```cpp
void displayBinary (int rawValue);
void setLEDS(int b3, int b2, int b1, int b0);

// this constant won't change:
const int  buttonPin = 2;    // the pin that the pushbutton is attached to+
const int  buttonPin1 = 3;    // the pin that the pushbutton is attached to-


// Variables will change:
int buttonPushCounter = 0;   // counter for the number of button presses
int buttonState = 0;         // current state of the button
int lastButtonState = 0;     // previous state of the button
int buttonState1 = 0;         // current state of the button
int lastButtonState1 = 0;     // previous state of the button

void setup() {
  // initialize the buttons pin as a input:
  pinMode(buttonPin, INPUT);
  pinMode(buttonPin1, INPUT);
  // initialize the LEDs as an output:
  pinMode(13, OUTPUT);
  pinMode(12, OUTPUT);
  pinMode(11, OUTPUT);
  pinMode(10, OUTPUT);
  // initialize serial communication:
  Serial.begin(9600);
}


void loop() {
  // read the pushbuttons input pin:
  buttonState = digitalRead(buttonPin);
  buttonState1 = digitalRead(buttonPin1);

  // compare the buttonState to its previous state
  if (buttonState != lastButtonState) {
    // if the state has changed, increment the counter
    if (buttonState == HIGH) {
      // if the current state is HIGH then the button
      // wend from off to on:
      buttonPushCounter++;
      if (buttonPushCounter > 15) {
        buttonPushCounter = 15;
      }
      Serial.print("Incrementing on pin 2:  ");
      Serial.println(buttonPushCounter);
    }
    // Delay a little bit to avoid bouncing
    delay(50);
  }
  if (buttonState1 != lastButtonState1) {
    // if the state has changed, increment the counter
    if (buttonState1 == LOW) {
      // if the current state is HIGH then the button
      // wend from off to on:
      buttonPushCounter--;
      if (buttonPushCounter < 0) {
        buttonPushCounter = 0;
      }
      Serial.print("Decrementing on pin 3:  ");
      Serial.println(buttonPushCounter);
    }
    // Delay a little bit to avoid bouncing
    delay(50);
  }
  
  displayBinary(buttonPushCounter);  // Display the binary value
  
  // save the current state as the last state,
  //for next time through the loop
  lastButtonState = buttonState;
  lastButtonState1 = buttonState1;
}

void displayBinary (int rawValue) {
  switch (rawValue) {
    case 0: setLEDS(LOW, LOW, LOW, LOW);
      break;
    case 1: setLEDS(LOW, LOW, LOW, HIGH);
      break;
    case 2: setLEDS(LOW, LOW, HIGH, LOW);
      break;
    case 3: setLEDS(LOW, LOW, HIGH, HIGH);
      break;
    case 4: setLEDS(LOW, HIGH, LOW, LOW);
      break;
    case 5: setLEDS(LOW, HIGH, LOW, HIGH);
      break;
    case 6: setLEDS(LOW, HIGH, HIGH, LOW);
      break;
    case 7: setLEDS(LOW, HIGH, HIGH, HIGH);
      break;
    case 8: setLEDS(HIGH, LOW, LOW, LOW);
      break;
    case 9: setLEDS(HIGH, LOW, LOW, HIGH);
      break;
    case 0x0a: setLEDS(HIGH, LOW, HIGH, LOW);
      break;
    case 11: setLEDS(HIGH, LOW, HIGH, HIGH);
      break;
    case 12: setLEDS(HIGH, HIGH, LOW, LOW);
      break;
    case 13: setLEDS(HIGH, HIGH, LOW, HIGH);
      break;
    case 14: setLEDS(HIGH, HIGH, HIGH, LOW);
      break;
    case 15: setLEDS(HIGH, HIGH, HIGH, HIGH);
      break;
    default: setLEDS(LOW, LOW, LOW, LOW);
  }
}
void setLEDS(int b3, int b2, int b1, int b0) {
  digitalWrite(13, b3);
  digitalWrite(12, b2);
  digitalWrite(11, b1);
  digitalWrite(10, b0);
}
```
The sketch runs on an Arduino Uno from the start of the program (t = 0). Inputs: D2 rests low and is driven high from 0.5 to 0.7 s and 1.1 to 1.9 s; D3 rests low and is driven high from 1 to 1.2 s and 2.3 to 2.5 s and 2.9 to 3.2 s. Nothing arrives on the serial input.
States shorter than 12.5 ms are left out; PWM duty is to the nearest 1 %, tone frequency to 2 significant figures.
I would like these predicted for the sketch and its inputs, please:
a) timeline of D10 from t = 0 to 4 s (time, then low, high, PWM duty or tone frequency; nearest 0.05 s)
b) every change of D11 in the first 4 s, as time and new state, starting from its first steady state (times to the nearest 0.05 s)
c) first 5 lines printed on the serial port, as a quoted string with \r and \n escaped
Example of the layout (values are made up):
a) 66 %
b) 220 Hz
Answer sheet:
a) 0 s low; 0.55 s high; 1.15 s low; 1.25 s high; 2.55 s low
b) 0 s low; 1.15 s high; 1.25 s low
c) "Incrementing on pin 2:  1\r\nIncrementing on pin 2:  2\r\nDecrementing on pin 3:  1\r\nDecrementing on pin 3:  0\r\nDecrementing on pin 3:  0\r\n"
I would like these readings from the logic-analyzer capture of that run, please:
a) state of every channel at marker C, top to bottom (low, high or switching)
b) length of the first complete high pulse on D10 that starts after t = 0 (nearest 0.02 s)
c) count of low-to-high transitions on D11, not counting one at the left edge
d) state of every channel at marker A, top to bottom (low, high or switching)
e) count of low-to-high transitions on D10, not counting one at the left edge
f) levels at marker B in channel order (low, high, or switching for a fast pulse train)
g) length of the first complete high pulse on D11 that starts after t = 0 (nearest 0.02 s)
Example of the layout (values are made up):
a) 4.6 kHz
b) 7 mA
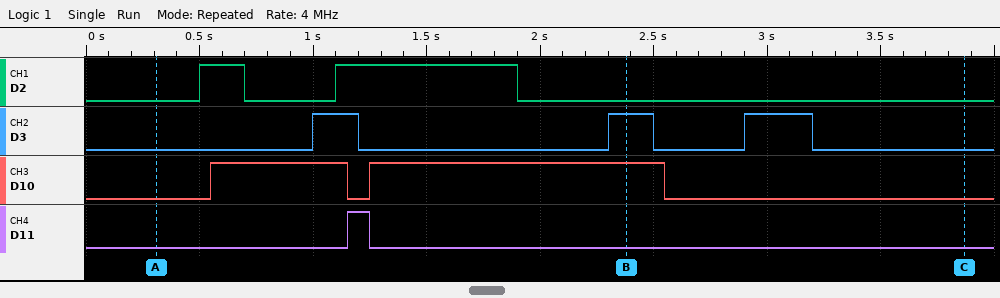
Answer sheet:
a) D2 low, D3 low, D10 low, D11 low
b) 0.60 s
c) 1
d) D2 low, D3 low, D10 low, D11 low
e) 2
f) D2 low, D3 high, D10 high, D11 low
g) 0.10 s
